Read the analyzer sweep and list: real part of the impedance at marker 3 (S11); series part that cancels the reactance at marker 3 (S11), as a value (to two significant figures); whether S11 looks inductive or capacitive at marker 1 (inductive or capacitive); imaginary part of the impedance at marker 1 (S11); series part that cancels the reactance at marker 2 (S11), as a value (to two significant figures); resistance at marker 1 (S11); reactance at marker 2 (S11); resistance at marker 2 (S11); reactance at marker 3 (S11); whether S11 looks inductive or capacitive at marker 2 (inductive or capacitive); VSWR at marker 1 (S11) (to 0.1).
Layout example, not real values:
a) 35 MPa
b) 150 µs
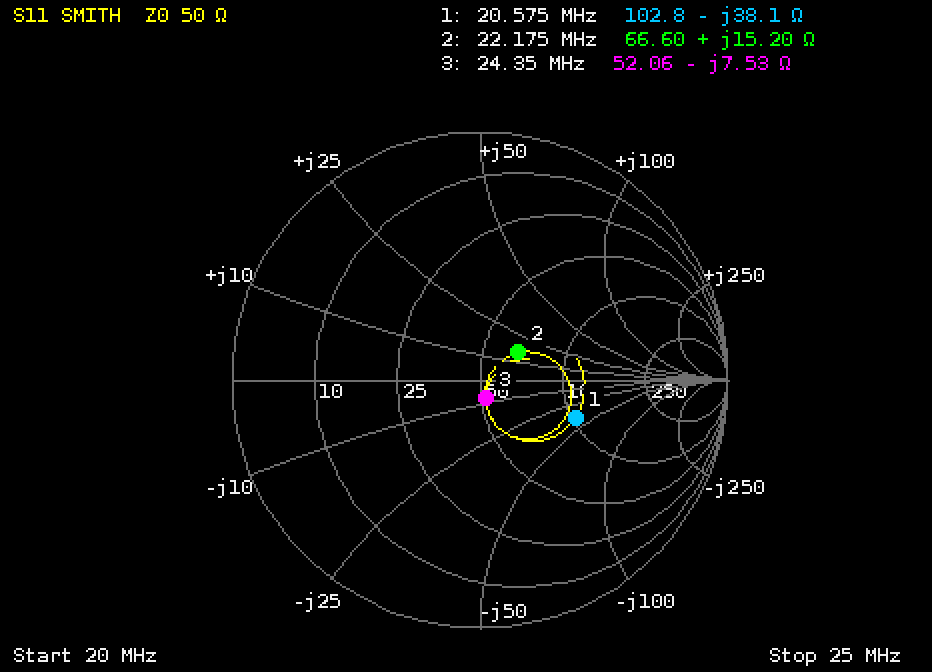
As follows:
a) 52.06 Ω
b) 49 nH
c) capacitive
d) -38.1 Ω
e) 470 pF
f) 102.8 Ω
g) +15.20 Ω
h) 66.60 Ω
i) -7.53 Ω
j) inductive
k) 2.4
